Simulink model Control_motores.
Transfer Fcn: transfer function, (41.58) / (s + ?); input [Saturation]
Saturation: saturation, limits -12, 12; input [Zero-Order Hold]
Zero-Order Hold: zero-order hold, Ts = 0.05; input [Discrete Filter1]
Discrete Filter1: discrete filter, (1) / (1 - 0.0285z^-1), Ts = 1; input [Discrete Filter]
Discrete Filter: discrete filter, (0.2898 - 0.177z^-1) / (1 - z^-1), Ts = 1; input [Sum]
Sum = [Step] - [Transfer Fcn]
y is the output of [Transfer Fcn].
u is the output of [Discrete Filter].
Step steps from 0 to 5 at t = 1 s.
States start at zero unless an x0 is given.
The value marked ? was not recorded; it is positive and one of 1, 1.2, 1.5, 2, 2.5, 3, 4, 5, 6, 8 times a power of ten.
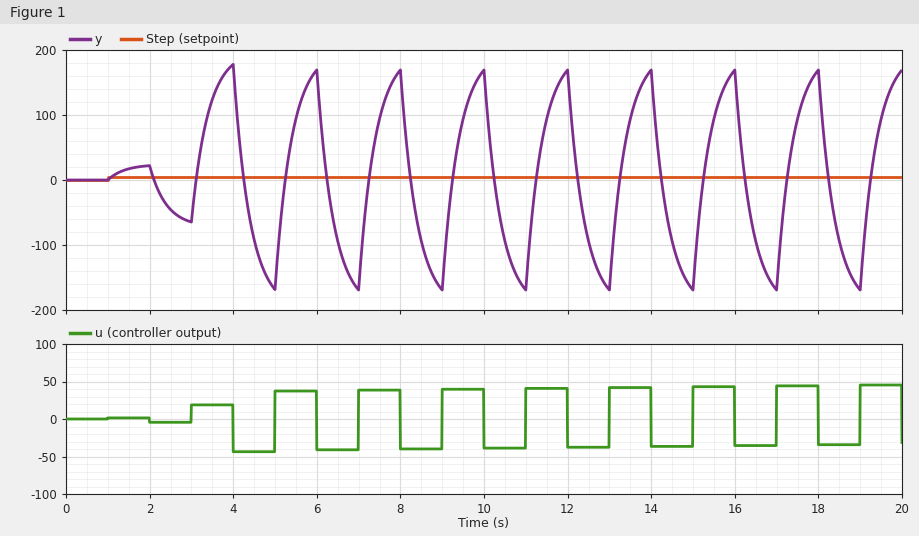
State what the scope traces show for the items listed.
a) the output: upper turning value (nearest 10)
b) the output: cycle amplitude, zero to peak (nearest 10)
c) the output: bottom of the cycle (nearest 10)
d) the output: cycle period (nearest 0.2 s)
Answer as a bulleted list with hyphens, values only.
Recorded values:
- 170
- 170
- -170
- 2.0 s
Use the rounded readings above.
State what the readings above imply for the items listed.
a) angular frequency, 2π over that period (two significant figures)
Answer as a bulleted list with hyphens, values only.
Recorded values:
- 3.1 rad/s
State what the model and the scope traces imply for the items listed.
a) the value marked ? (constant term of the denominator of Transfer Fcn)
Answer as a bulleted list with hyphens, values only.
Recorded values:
- 2.5
